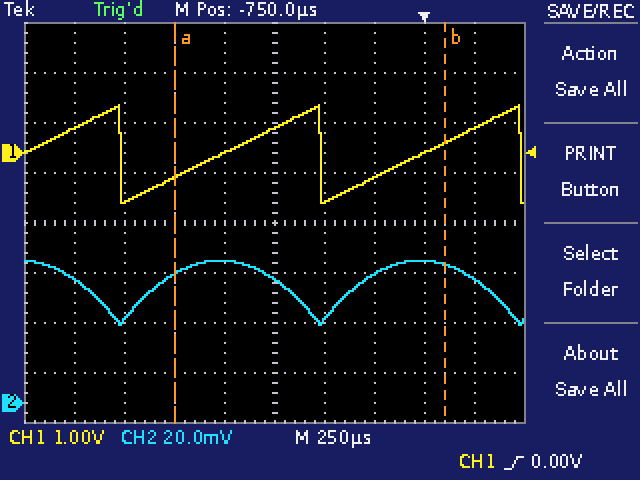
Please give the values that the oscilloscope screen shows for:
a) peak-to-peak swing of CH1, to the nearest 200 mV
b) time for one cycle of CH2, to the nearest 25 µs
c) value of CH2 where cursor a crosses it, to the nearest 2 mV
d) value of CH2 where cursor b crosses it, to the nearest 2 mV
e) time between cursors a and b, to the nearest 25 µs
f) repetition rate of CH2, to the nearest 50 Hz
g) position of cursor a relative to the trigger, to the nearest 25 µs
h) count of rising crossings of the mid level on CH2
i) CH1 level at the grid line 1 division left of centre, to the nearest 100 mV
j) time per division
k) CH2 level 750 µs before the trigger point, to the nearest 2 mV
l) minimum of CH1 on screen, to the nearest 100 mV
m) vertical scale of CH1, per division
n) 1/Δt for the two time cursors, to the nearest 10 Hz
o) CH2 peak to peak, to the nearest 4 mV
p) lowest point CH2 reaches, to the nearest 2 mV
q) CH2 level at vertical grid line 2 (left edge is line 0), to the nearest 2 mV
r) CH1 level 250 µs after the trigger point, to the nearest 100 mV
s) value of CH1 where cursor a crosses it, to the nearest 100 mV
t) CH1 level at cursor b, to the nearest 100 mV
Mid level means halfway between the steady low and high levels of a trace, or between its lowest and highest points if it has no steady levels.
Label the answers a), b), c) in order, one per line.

a) 2.0 V
b) 1.000 ms
c) 52 mV
d) 56 mV
e) 1.350 ms
f) 1.00 kHz
g) -1.250 ms
h) 2
i) 0.0 V
j) 250 µs
k) 50 mV
l) -1.0 V
m) 1 V
n) 740 Hz
o) 24 mV
p) 32 mV
q) 34 mV
r) 500 mV
s) -500 mV
t) 200 mV
